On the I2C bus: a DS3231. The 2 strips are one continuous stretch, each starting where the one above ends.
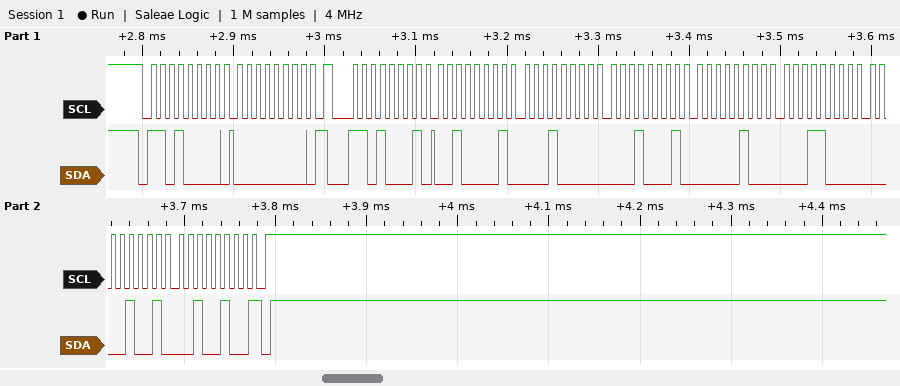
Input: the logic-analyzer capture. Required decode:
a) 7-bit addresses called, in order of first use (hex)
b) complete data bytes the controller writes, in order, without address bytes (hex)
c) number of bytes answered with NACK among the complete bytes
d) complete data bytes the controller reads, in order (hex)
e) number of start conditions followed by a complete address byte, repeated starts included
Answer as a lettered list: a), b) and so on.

a) 0x68
b) 00
c) 1
d) 21 10 11 04 18 09 24
e) 2
